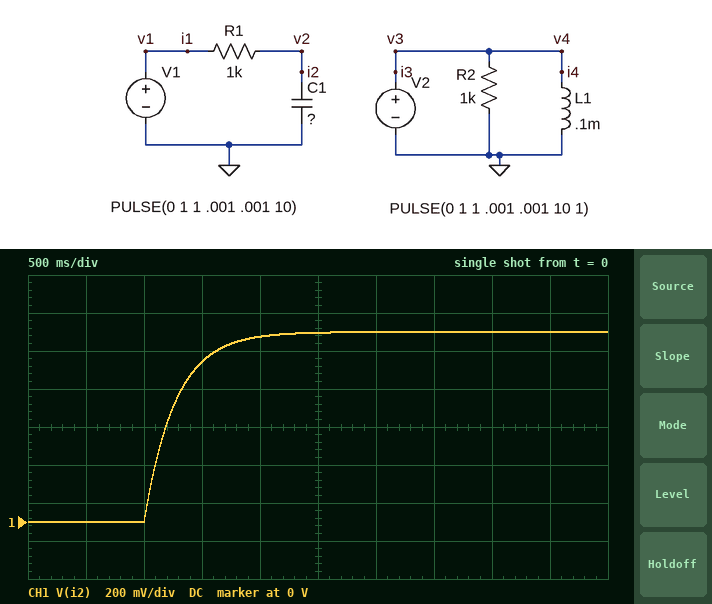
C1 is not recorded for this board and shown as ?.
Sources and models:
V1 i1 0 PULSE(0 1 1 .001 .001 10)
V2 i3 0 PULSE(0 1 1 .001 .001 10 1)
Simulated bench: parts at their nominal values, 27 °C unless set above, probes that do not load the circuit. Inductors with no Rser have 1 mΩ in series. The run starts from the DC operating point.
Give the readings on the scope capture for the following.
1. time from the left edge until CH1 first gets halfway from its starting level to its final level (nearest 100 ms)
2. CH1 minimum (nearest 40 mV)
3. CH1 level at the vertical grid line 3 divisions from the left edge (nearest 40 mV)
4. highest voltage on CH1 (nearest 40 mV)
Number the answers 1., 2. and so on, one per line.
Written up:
1. 1.2 s
2. 0 V
3. 840 mV
4. 1.00 V
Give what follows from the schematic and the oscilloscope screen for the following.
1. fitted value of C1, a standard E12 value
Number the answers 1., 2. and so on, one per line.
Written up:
1. 270 µF
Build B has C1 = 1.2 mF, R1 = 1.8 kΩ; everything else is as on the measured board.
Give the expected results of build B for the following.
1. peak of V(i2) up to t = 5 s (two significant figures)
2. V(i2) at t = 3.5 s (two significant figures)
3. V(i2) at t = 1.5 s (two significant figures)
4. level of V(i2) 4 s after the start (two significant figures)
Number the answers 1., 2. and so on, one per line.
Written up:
1. 840 mV
2. 690 mV
3. 210 mV
4. 750 mV
